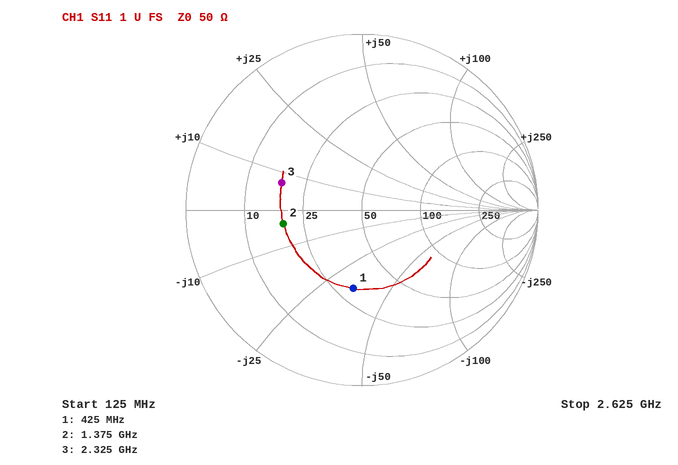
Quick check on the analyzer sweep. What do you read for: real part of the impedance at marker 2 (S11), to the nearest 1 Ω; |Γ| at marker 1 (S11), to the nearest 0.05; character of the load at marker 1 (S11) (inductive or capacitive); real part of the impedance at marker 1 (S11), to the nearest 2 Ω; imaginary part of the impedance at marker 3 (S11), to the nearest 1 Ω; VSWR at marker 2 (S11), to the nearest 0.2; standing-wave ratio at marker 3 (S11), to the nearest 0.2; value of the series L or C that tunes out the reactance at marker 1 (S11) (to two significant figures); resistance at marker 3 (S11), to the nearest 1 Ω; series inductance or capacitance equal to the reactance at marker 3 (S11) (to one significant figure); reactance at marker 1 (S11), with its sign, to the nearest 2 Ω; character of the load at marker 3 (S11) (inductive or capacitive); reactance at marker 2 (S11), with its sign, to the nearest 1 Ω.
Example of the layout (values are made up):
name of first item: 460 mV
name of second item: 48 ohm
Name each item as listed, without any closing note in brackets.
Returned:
real part of the impedance at marker 2 (S11), to the nearest 1 Ω: 19 Ω
|Γ| at marker 1 (S11), to the nearest 0.05: 0.45
character of the load at marker 1 (S11): capacitive
real part of the impedance at marker 1 (S11), to the nearest 2 Ω: 30 Ω
imaginary part of the impedance at marker 3 (S11), to the nearest 1 Ω: +7 Ω
VSWR at marker 2 (S11), to the nearest 0.2: 2.6
standing-wave ratio at marker 3 (S11), to the nearest 0.2: 2.8
value of the series L or C that tunes out the reactance at marker 1 (S11): 13 nH
resistance at marker 3 (S11), to the nearest 1 Ω: 18 Ω
series inductance or capacitance equal to the reactance at marker 3 (S11): 500 pH
reactance at marker 1 (S11), with its sign, to the nearest 2 Ω: -34 Ω
character of the load at marker 3 (S11): inductive
reactance at marker 2 (S11), with its sign, to the nearest 1 Ω: -4 Ω
